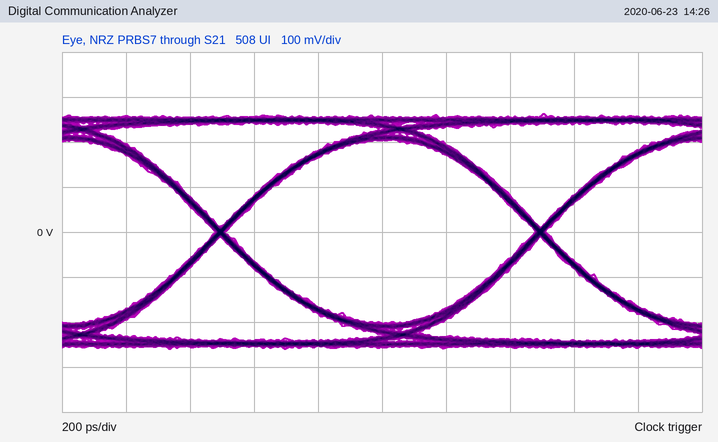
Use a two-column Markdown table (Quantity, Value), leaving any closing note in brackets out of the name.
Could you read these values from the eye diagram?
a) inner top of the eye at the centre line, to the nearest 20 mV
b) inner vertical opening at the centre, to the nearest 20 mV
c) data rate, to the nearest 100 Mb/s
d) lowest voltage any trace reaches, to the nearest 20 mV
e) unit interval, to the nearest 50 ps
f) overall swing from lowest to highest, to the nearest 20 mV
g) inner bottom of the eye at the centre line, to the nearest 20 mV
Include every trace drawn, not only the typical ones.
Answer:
| Quantity | Value |
|---|---|
| inner top of the eye at the centre line, to the nearest 20 mV | 200 mV |
| inner vertical opening at the centre, to the nearest 20 mV | 400 mV |
| data rate, to the nearest 100 Mb/s | 1.0 Gb/s |
| lowest voltage any trace reaches, to the nearest 20 mV | -260 mV |
| unit interval, to the nearest 50 ps | 1.00 ns |
| overall swing from lowest to highest, to the nearest 20 mV | 520 mV |
| inner bottom of the eye at the centre line, to the nearest 20 mV | -200 mV |
